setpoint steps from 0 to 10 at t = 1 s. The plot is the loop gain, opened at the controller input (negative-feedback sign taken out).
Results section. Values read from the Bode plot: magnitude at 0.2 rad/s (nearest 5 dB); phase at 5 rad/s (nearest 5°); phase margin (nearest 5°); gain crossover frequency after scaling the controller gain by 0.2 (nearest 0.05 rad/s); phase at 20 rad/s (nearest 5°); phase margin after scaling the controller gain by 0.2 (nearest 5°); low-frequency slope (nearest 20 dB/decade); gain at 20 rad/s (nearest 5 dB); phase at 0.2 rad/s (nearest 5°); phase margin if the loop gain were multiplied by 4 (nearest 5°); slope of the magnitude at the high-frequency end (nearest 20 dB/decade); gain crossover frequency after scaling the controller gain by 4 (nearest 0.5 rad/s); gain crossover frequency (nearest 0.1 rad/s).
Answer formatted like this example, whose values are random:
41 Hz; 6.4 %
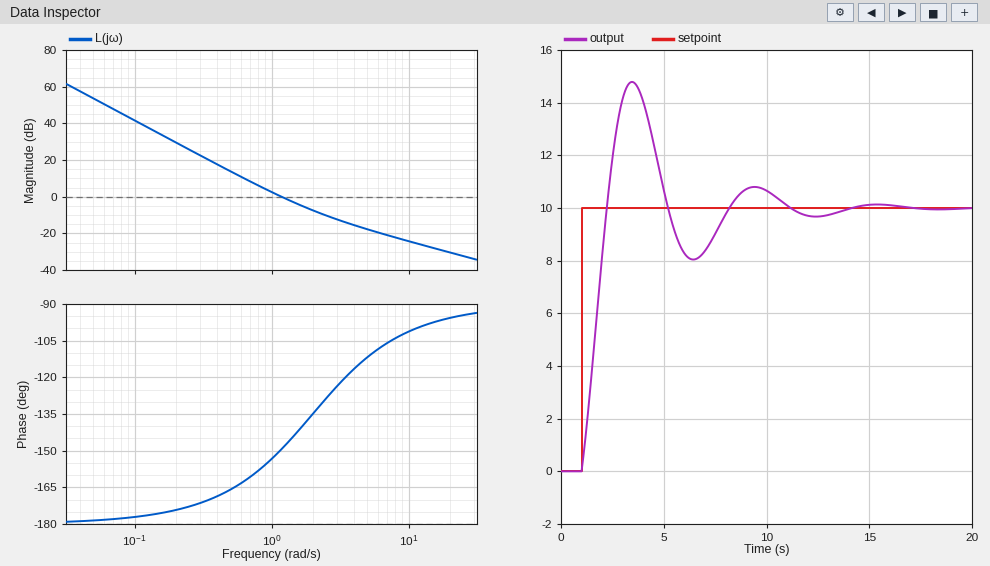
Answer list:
30 dB; -110°; 30°; 0.50 rad/s; -95°; 15°; -40 dB/decade; -30 dB; -175°; 55°; -20 dB/decade; 3.0 rad/s; 1.2 rad/s
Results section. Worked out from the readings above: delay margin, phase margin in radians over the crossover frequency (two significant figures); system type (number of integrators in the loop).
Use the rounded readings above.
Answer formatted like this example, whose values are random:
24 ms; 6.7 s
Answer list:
0.44 s; 2
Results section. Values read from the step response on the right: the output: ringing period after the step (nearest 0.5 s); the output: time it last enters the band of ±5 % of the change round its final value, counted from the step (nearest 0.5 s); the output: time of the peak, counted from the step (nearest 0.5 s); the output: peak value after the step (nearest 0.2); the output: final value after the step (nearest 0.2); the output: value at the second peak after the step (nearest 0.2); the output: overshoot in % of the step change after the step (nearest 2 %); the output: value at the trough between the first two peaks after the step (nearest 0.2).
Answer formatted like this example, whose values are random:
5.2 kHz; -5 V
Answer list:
6.0 s; 9.5 s; 2.5 s; 14.8; 10.0; 10.8; 48 %; 8.0
